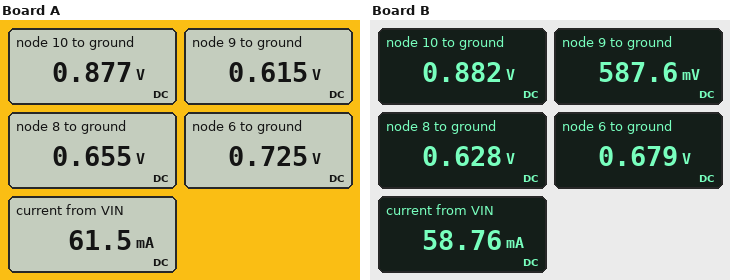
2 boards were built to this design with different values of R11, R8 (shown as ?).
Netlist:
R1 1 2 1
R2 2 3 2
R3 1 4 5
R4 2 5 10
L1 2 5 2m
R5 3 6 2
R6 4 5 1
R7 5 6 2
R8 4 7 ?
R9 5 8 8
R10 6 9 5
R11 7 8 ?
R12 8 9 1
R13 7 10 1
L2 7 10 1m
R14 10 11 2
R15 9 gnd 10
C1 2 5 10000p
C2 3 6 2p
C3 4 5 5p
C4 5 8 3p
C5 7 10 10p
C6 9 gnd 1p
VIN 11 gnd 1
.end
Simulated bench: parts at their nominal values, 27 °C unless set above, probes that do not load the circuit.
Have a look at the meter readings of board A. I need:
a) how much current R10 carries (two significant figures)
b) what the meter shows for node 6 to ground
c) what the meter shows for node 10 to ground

22 mA
0.725 V
0.877 V
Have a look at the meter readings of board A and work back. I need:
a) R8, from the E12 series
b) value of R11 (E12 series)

2.7 Ω
8.2 Ω
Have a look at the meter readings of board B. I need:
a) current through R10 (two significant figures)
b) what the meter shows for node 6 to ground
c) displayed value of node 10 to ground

18 mA
0.679 V
0.882 V
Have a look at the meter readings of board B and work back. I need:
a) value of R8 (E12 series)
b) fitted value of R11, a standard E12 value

5.6 Ω
8.2 Ω
